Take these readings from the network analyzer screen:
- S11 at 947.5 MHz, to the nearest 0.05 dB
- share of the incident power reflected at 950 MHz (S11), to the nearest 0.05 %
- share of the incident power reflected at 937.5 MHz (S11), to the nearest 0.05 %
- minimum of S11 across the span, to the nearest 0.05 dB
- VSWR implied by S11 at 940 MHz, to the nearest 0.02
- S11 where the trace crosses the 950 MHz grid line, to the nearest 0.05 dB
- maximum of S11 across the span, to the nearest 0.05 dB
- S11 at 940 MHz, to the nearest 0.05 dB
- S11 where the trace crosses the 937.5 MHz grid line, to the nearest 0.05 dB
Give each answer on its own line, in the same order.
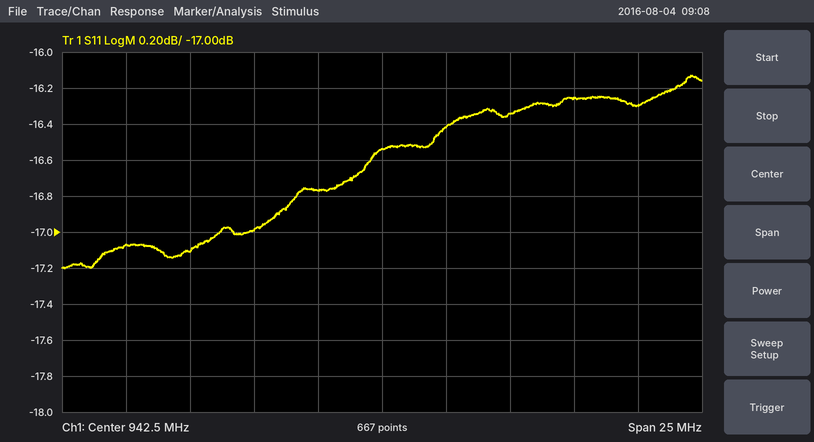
-16.35 dB
2.35 %
2.00 %
-17.20 dB
1.34
-16.25 dB
-16.15 dB
-16.75 dB
-17.00 dB
